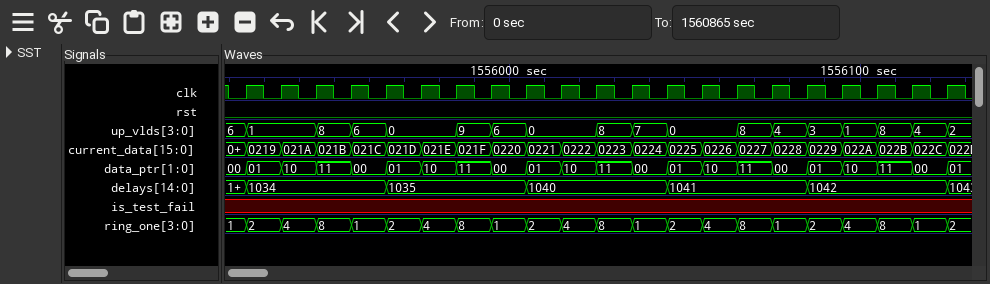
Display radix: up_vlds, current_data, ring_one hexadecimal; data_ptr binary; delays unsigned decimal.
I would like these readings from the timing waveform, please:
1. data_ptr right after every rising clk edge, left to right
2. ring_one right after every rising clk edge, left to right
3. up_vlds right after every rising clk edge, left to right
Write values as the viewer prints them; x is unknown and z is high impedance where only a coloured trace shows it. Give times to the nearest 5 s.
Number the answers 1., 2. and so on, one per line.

1. 01, 10, 11, 00, 01, 10, 11, 00, 01, 10, 11, 00, 01, 10, 11, 00, 01, 10, 11, 00, 01
2. 2, 4, 8, 1, 2, 4, 8, 1, 2, 4, 8, 1, 2, 4, 8, 1, 2, 4, 8, 1, 2
3. 1, 1, 8, 6, 0, 0, 9, 6, 0, 0, 8, 7, 0, 0, 8, 4, 3, 1, 8, 4, 2
